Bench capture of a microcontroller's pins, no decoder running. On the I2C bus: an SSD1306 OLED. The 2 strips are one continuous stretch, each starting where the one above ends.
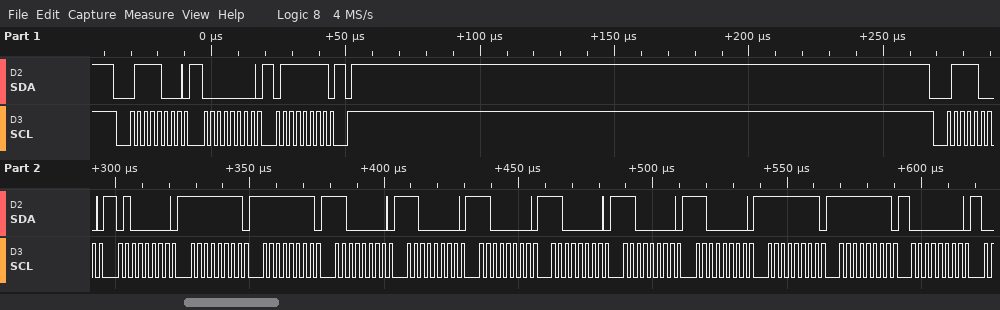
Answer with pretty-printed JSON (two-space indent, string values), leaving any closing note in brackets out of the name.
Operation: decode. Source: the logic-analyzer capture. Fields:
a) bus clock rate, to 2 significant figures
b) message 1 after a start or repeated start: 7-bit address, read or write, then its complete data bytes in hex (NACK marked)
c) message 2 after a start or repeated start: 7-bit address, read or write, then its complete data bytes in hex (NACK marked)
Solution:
{
  "bus clock rate, to 2 significant figures": "400 kHz",
  "message 1 after a start or repeated start: 7-bit address, read or write, then its complete data bytes in hex": "0x3C write: 00 7F",
  "message 2 after a start or repeated start: 7-bit address, read or write, then its complete data bytes in hex": "0x3C write: 40 FF FF C0 C0 C0 C0 C0 C0 FF FF 00"
}
